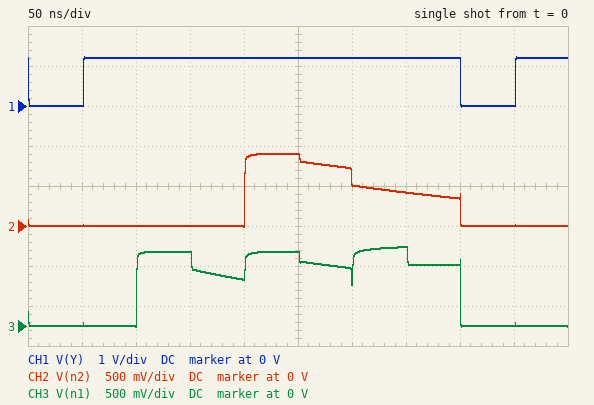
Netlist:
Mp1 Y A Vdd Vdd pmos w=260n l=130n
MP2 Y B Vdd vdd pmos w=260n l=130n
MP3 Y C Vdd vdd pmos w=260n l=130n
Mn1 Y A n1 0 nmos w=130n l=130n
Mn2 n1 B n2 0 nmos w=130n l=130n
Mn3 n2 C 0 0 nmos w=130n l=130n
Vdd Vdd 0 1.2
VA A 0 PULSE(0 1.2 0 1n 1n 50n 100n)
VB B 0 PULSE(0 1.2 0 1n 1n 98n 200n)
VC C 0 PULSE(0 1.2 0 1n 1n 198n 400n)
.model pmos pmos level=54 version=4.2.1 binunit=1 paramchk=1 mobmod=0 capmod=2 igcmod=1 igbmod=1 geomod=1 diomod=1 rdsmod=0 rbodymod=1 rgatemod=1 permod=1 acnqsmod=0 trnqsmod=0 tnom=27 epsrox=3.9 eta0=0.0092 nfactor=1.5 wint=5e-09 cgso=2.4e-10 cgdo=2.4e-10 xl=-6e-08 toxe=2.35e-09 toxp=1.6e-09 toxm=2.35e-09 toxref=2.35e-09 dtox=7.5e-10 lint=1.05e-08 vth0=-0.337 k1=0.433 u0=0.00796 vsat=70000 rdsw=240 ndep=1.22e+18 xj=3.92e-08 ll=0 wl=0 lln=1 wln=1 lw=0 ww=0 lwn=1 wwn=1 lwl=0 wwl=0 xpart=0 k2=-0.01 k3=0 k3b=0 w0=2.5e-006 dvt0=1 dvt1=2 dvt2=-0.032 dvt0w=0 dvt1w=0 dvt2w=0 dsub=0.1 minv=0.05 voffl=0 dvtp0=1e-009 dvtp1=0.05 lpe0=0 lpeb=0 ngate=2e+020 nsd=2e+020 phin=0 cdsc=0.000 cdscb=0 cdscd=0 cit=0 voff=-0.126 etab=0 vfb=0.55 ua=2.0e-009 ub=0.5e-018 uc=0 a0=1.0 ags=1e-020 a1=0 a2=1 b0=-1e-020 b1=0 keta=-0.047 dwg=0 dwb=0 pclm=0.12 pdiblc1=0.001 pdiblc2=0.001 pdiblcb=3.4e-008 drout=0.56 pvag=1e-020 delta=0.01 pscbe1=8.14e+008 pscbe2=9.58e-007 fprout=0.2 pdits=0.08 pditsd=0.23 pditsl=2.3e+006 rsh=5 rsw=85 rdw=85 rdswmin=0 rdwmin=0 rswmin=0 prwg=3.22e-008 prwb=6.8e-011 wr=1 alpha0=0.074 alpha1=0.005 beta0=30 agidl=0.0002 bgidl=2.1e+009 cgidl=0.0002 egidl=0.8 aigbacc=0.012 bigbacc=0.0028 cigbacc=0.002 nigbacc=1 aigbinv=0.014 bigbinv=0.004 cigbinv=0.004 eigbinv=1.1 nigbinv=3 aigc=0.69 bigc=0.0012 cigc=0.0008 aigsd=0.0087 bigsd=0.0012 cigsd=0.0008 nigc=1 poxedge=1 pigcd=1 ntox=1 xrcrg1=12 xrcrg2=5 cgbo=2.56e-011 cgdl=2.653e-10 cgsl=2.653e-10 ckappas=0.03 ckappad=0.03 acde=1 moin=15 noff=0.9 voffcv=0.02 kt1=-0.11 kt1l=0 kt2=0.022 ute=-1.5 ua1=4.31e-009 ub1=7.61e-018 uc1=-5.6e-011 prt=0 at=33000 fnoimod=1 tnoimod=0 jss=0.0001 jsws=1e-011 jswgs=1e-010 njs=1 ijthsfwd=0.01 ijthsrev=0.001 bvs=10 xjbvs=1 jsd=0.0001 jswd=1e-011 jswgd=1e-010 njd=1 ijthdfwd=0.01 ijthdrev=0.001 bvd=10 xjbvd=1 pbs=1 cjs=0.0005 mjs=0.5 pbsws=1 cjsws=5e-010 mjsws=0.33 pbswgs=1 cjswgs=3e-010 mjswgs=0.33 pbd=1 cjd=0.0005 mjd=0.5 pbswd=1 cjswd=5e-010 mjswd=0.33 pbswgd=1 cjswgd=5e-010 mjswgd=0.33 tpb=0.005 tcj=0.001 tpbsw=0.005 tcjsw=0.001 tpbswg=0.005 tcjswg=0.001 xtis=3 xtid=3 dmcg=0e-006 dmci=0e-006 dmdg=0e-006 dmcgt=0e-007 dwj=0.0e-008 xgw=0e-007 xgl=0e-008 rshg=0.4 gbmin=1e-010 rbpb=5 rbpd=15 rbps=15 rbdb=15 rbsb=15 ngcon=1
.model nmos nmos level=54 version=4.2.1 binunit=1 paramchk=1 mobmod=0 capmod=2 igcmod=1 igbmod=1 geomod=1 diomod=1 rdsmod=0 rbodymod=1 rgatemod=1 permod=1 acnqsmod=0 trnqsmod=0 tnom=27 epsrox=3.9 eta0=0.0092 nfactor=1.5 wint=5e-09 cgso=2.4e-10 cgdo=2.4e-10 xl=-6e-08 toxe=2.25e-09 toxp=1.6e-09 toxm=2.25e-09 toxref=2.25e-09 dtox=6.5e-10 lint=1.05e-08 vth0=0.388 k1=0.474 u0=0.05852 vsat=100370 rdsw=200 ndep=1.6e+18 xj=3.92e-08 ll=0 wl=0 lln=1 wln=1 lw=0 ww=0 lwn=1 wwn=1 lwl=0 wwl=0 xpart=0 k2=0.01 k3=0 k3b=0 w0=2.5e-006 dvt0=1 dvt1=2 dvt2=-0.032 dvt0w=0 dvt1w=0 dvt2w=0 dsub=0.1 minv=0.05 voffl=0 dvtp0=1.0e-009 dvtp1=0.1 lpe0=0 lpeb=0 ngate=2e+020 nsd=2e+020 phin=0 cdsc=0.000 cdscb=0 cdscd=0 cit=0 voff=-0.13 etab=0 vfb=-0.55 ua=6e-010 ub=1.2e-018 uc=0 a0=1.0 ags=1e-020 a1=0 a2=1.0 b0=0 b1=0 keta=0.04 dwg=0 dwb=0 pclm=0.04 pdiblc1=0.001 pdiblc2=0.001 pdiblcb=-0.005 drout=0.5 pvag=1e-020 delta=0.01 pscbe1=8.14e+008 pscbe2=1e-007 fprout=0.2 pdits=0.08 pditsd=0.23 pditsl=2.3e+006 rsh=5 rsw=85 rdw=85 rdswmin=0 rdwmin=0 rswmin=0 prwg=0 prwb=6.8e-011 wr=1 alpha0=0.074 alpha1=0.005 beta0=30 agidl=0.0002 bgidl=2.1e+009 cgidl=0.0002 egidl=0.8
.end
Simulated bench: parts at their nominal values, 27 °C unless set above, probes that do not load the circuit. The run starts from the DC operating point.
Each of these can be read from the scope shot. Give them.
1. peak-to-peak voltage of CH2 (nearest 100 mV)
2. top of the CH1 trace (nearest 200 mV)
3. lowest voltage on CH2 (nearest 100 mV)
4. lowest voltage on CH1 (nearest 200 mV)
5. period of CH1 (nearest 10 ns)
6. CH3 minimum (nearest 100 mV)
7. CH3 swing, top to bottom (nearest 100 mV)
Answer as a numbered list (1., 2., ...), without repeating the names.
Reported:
1. 900 mV
2. 1.2 V
3. 0 V
4. 0 V
5. 400 ns
6. 0 V
7. 1.0 V
